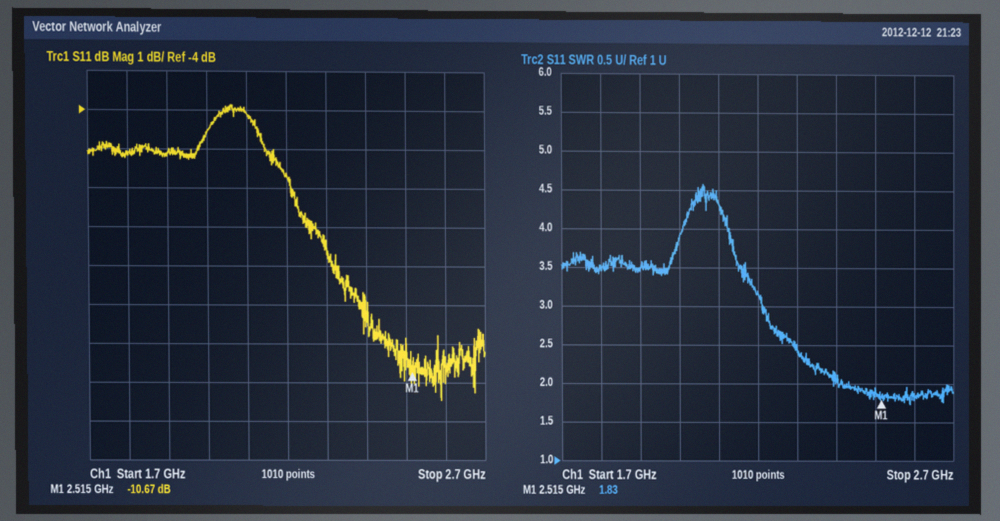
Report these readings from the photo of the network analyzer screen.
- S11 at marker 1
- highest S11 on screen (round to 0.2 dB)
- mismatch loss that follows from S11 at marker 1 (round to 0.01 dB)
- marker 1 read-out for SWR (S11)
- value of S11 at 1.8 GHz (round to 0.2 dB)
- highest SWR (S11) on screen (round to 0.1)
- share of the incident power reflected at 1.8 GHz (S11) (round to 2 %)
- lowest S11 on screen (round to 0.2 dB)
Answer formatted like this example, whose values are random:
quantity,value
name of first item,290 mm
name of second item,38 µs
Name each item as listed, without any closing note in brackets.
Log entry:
quantity,value
S11 at marker 1,-10.67 dB
highest S11 on screen,-3.8 dB
mismatch loss that follows from S11 at marker 1,0.39 dB
marker 1 read-out for SWR,1.83
value of S11 at 1.8 GHz,-5.2 dB
highest SWR (S11) on screen,4.6
share of the incident power reflected at 1.8 GHz (S11),30 %
lowest S11 on screen,-11.4 dB
